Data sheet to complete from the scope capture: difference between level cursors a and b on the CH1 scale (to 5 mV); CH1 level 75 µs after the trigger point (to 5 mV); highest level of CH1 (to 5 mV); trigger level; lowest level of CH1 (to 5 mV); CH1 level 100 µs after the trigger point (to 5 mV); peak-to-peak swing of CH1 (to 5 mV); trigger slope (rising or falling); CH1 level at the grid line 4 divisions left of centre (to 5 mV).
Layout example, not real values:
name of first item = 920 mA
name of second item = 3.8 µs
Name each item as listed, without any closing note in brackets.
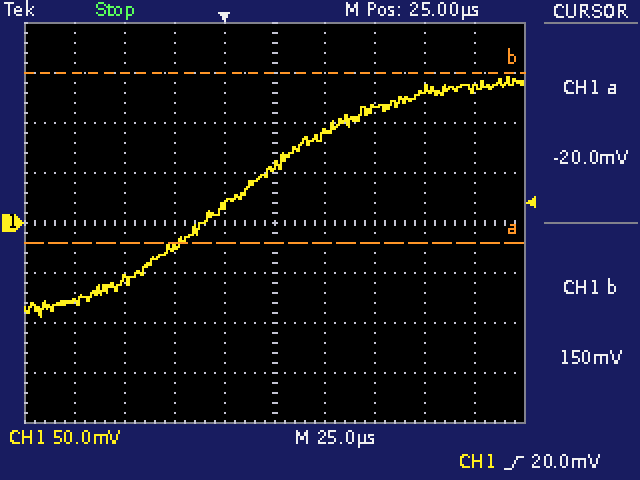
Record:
difference between level cursors a and b on the CH1 scale = 170 mV
CH1 level 75 µs after the trigger point = 115 mV
highest level of CH1 = 145 mV
trigger level = 20.0 mV
lowest level of CH1 = -95 mV
CH1 level 100 µs after the trigger point = 135 mV
peak-to-peak swing of CH1 = 240 mV
trigger slope = rising
CH1 level at the grid line 4 divisions left of centre = -80 mV
